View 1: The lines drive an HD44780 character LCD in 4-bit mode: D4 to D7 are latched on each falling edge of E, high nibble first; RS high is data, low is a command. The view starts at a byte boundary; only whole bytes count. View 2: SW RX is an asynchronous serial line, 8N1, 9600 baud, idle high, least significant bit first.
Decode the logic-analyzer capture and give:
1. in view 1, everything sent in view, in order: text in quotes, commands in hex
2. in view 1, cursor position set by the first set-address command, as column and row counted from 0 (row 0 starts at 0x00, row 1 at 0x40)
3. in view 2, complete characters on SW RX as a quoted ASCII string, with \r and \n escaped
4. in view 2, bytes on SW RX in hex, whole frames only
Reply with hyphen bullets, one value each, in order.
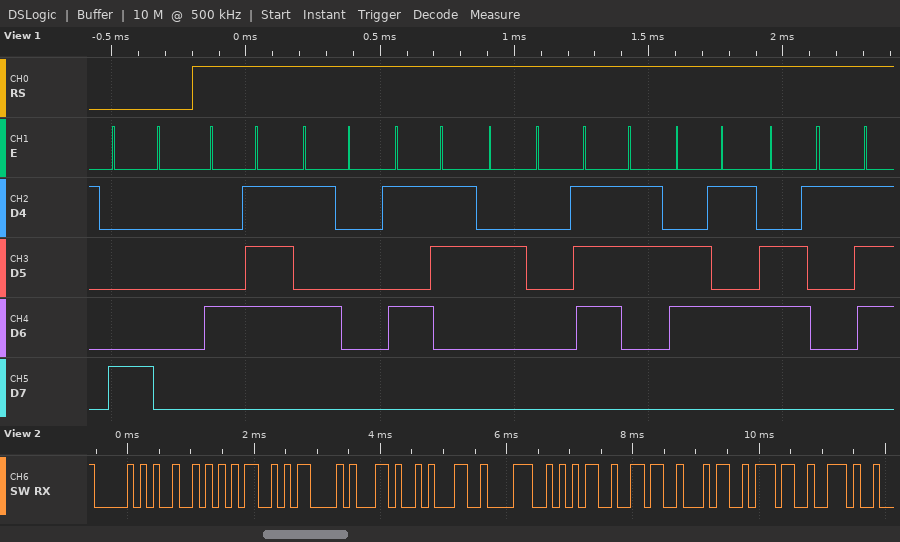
- 0x80 "GPS sea"
- column 0, row 0
- "PRMC,185647."
- 0x50 0x52 0x4D 0x43 0x2C 0x31 0x38 0x35 0x36 0x34 0x37 0x2E
